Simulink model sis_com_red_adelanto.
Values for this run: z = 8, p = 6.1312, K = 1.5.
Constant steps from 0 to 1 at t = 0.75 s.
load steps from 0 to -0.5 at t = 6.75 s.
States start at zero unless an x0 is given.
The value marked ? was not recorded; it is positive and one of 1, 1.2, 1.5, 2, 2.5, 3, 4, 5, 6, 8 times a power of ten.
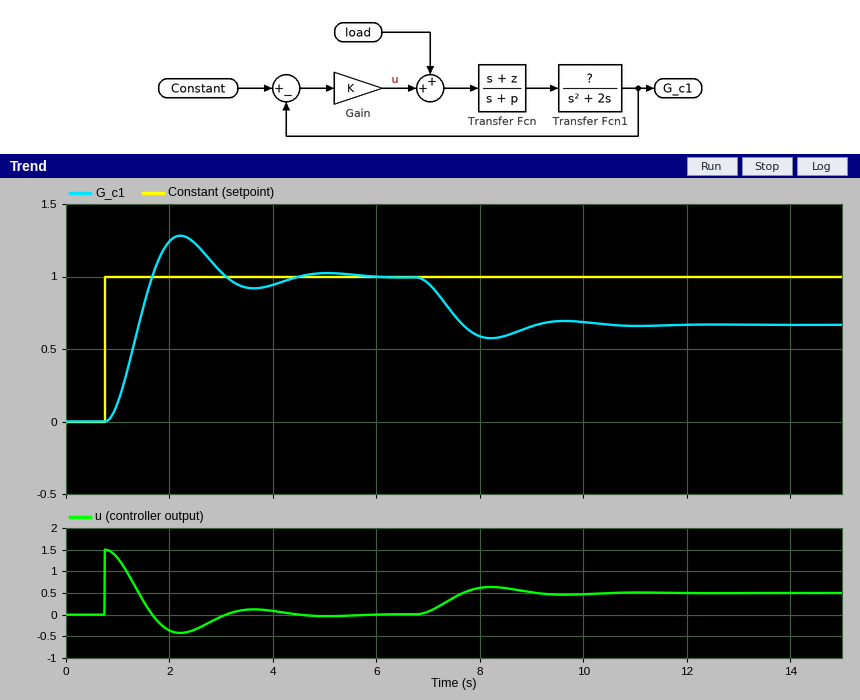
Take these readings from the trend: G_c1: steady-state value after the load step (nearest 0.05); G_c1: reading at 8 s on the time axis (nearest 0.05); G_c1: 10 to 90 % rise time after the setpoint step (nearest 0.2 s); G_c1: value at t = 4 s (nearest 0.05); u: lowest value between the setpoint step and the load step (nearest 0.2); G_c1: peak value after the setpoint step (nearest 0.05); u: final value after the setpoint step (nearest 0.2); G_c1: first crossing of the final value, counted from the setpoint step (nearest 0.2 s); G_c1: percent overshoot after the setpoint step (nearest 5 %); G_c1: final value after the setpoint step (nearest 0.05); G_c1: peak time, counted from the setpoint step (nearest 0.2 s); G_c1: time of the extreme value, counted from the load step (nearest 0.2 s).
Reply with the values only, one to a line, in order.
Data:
0.65
0.60
0.6 s
0.95
-0.4
1.30
0.0
1.0 s
30 %
1.00
1.4 s
1.4 s
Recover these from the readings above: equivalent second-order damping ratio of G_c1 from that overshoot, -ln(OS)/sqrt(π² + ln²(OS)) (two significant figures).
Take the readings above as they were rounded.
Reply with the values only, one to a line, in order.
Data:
0.36
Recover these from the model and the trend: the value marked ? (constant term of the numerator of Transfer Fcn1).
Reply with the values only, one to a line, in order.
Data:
3
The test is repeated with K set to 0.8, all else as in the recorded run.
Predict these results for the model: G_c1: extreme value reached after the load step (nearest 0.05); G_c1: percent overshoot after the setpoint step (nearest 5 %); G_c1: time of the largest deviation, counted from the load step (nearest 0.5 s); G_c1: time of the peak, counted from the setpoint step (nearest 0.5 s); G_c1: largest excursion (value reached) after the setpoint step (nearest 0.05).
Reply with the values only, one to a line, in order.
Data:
0.30
15 %
2.0 s
2.0 s
1.15
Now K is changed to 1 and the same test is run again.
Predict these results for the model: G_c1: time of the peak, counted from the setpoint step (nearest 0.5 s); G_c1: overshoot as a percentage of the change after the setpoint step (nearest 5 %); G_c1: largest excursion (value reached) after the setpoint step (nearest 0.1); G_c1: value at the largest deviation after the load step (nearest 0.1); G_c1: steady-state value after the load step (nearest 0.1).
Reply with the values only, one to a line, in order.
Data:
2.0 s
20 %
1.2
0.4
0.5
